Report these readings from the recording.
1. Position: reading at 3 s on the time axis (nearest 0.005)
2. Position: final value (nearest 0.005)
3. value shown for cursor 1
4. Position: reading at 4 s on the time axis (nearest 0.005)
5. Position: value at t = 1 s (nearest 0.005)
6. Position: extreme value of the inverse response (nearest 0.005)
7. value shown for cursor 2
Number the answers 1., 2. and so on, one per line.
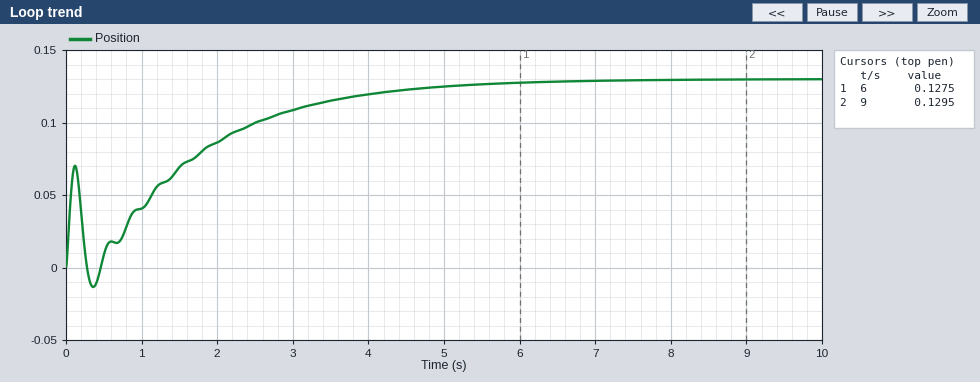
1. 0.110
2. 0.130
3. 0.1275
4. 0.120
5. 0.040
6. -0.015
7. 0.1295
